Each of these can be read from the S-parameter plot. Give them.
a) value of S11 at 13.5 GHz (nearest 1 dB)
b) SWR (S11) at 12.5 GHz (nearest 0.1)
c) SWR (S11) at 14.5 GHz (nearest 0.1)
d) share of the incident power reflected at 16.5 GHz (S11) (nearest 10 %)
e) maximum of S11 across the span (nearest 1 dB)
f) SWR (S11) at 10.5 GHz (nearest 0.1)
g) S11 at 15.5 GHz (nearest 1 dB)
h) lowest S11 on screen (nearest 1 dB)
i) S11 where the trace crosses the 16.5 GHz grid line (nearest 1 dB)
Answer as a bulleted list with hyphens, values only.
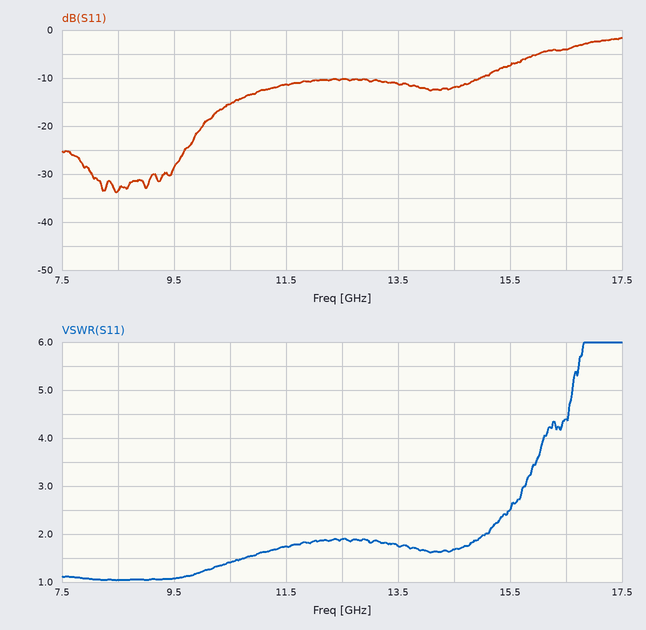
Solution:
- -11 dB
- 1.9
- 1.7
- 40 %
- -2 dB
- 1.4
- -7 dB
- -34 dB
- -4 dB
